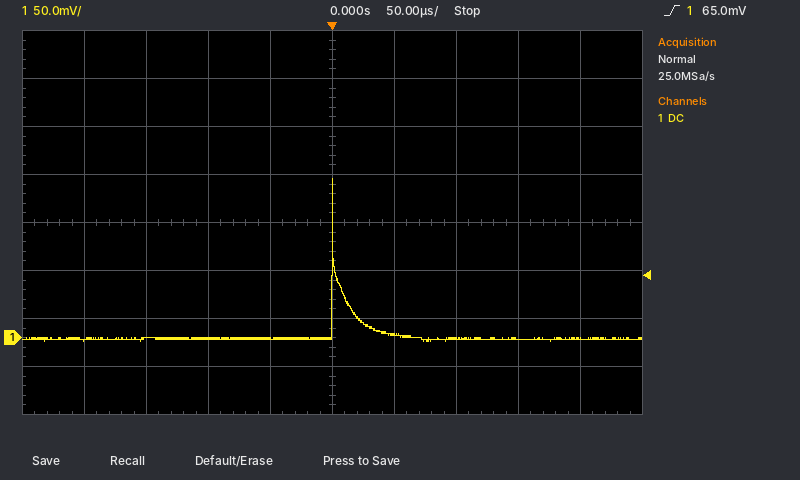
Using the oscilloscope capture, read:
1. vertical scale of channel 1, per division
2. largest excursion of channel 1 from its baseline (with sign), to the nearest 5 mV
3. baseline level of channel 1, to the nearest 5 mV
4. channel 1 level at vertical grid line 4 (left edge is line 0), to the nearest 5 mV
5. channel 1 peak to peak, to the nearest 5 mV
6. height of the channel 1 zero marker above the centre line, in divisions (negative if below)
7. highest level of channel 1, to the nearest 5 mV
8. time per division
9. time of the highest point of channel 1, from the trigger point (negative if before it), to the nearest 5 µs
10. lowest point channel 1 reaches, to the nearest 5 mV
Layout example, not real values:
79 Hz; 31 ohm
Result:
50 mV; +165 mV; 0 mV; 0 mV; 170 mV; -2.4 div; 165 mV; 50 µs; 0 µs; -5 mV
